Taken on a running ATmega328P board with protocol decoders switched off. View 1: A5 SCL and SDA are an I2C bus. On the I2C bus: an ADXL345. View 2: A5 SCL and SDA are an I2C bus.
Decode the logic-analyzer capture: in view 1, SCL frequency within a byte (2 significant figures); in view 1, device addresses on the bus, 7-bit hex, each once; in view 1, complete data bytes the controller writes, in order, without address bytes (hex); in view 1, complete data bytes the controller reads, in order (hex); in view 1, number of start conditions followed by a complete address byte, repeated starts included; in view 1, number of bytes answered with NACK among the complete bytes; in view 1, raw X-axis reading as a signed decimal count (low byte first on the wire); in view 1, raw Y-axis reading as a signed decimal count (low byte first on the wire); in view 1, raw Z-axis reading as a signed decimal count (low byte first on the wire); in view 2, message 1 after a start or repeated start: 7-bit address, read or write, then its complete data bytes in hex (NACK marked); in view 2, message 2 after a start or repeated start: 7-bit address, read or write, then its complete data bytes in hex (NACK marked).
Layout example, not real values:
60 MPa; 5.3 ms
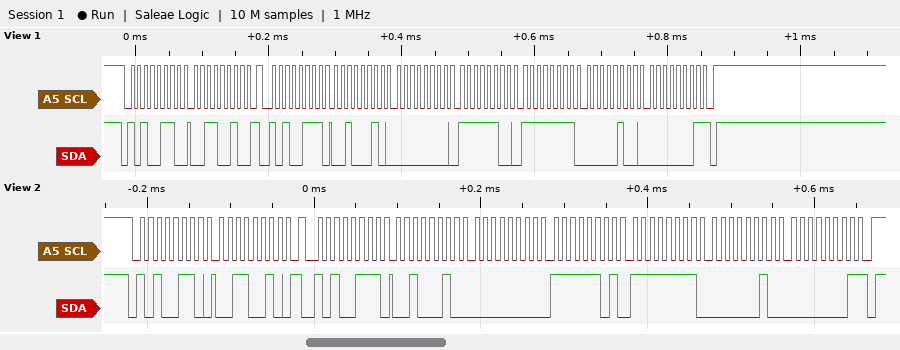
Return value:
100 kHz; 0x53; 32; 22 00 FC FF 04 01; 2; 1; 34; -4; 260; 0x53 write: 32; 0x53 read: 22 00 FD FF 02 01 NACK
